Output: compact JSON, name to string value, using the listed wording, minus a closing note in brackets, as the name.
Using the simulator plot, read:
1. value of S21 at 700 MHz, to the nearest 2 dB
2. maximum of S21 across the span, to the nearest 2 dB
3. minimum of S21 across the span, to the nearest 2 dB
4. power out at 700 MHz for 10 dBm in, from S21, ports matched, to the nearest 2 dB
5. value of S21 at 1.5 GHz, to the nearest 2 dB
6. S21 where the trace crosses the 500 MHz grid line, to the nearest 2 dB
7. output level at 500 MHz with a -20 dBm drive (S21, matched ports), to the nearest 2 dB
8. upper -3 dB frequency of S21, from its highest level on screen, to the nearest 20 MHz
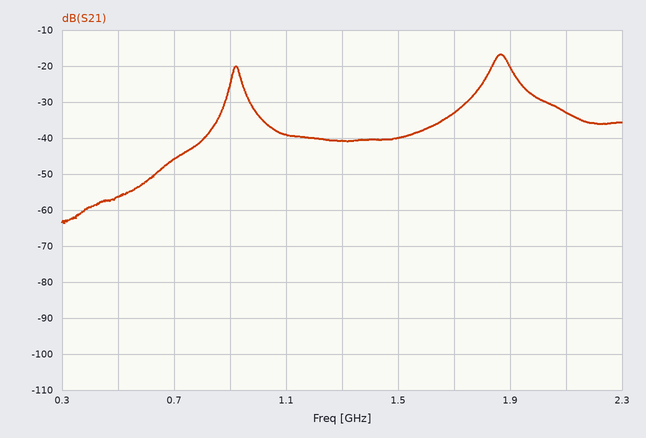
{"value of S21 at 700 MHz, to the nearest 2 dB": "-46 dB", "maximum of S21 across the span, to the nearest 2 dB": "-16 dB", "minimum of S21 across the span, to the nearest 2 dB": "-64 dB", "power out at 700 MHz for 10 dBm in, from S21, ports matched, to the nearest 2 dB": "-36 dBm", "value of S21 at 1.5 GHz, to the nearest 2 dB": "-40 dB", "S21 where the trace crosses the 500 MHz grid line, to the nearest 2 dB": "-56 dB", "output level at 500 MHz with a -20 dBm drive (S21, matched ports), to the nearest 2 dB": "-76 dBm", "upper -3 dB frequency of S21, from its highest level on screen, to the nearest 20 MHz": "1.90 GHz"}
